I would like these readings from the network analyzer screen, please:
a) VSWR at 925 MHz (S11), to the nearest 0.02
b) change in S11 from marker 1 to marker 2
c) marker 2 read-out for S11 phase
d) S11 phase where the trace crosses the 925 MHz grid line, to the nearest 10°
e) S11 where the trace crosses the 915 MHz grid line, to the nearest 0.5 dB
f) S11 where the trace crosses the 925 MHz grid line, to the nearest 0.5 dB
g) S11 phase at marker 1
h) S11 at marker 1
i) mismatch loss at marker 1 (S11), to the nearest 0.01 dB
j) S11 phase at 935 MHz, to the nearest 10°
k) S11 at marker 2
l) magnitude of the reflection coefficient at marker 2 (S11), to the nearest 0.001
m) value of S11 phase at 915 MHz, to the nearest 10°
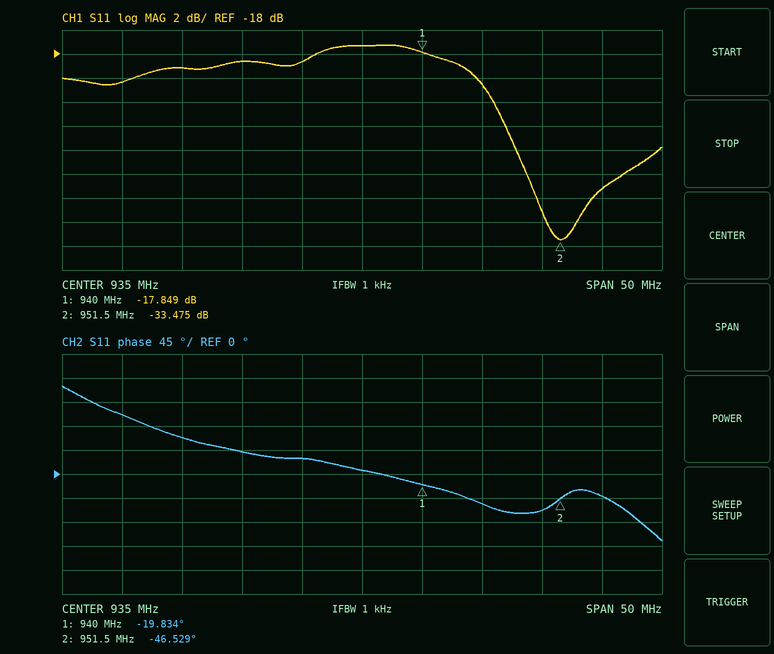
1.26
-15.626 dB
-46.529°
40°
-20.5 dB
-18.5 dB
-19.834°
-17.849 dB
0.07 dB
10°
-33.475 dB
0.021
110°
